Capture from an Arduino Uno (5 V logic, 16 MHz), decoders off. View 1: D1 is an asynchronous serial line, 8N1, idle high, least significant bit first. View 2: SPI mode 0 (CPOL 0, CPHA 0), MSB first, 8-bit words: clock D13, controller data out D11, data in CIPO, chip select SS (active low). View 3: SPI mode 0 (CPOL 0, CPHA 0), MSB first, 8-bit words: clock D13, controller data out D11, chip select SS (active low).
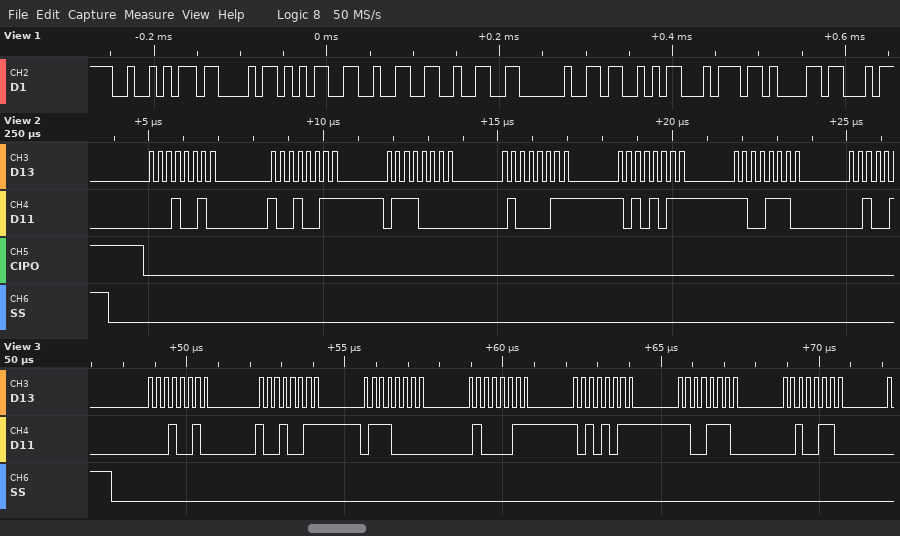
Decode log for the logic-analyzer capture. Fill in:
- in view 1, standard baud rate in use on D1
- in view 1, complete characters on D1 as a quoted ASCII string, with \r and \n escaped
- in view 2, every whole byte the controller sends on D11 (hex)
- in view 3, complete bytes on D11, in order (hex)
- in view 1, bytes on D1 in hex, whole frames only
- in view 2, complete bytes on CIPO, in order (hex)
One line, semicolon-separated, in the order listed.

115200 baud; "RC522 Sta"; 12 93 70 43 AB CE; 0x12 0x93 0x70 0x43 0xAB 0xCE 0x26; 52 43 35 32 32 20 53 74 61; 00 00 00 00 00 00
